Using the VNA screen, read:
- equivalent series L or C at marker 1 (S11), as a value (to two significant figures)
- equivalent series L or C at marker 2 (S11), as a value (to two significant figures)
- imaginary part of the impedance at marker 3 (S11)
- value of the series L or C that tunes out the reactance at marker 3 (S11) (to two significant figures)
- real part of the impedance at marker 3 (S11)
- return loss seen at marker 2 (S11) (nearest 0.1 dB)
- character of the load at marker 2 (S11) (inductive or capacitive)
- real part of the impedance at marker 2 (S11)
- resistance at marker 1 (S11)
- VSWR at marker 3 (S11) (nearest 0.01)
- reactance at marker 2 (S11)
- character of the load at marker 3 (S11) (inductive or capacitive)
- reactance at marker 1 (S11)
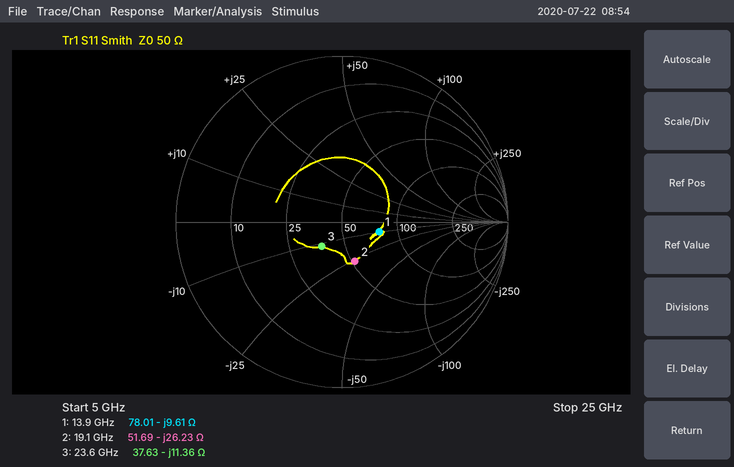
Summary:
1.2 pF
320 fF
-11.36 Ω
77 pH
37.63 Ω
12.0 dB
capacitive
51.69 Ω
78.01 Ω
1.47
-26.23 Ω
capacitive
-9.61 Ω
